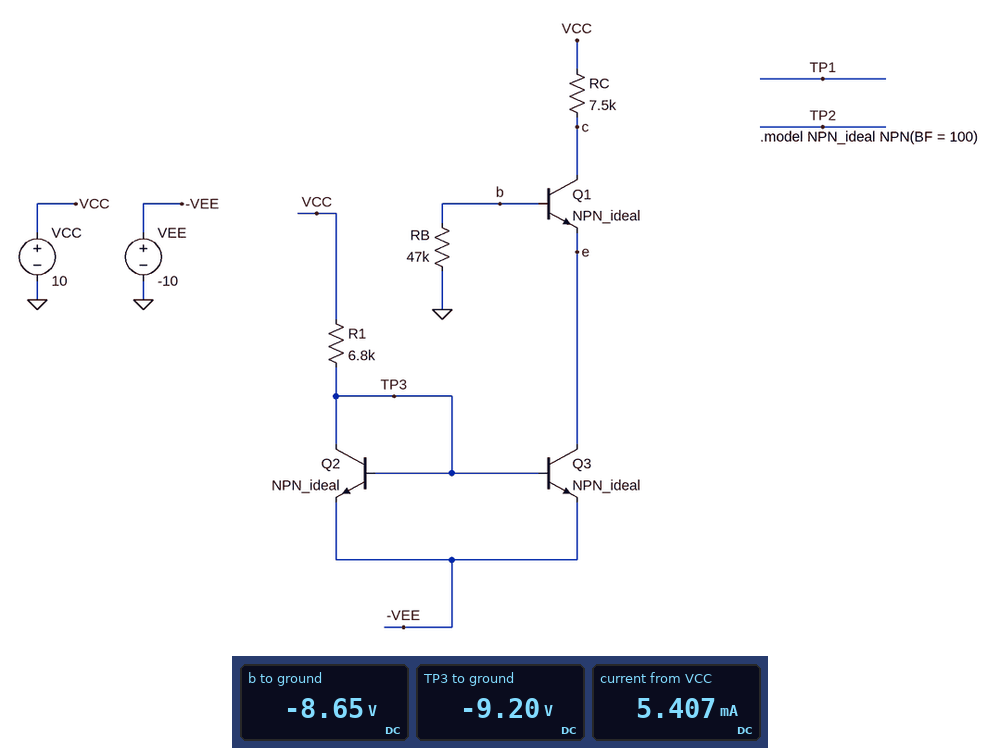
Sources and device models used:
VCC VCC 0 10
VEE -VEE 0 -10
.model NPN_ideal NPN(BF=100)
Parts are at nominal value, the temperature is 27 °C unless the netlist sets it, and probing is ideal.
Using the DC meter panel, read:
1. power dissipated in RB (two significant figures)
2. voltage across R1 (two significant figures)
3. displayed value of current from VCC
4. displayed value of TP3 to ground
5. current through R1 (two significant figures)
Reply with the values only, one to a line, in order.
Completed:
1.6 mW
19 V
5.407 mA
-9.20 V
2.8 mA
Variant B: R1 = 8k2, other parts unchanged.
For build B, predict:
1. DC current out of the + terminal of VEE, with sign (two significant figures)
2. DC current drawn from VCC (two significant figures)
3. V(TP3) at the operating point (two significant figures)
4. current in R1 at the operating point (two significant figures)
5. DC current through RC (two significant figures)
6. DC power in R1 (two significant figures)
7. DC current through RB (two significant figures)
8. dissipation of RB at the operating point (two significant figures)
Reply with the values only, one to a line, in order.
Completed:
-4.6 mA
4.5 mA
-9.2 V
2.3 mA
2.2 mA
45 mW
120 µA
670 µW
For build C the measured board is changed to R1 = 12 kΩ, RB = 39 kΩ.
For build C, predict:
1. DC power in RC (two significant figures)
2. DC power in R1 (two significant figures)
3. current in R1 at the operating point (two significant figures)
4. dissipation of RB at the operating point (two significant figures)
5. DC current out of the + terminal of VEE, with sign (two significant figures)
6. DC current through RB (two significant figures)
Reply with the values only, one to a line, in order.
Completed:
18 mW
31 mW
1.6 mA
23 µW
-3.2 mA
24 µA
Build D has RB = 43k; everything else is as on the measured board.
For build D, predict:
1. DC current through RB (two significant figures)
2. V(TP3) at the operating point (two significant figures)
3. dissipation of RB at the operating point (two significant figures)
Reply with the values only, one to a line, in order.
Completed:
200 µA
-9.2 V
1.7 mW
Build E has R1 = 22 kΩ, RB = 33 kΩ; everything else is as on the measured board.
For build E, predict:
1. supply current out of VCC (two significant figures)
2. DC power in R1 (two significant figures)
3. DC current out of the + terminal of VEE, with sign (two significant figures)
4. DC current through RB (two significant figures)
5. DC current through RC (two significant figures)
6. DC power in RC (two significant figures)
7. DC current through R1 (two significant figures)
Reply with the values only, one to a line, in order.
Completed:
1.7 mA
17 mW
-1.7 mA
8.5 µA
850 µA
5.4 mW
870 µA
